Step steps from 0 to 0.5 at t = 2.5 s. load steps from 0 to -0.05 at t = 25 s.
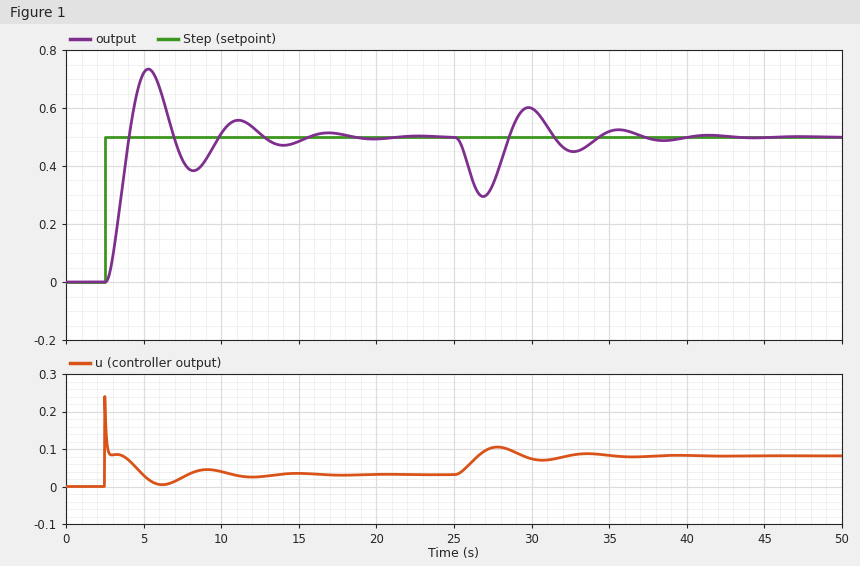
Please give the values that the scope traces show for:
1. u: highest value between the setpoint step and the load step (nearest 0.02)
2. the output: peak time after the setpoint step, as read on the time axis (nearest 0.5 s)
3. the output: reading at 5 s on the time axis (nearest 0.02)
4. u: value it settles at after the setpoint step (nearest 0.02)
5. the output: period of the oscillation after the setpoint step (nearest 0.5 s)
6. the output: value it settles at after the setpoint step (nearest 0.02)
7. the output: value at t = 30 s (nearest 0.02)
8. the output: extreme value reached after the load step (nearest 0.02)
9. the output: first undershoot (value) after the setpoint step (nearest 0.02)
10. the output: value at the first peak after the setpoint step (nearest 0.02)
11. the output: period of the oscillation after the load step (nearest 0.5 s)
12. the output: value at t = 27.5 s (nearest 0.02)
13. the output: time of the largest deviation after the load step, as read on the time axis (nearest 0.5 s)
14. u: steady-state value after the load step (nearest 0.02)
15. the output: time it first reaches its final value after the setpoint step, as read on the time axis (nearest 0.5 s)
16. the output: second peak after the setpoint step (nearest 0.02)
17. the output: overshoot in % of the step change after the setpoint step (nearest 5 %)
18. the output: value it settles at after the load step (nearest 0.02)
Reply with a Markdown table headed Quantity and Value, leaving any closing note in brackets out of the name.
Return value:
| Quantity | Value |
|---|---|
| u: highest value between the setpoint step and the load step | 0.24 |
| the output: peak time after the setpoint step, as read on the time axis | 5.5 s |
| the output: reading at 5 s on the time axis | 0.72 |
| u: value it settles at after the setpoint step | 0.04 |
| the output: period of the oscillation after the setpoint step | 6.0 s |
| the output: value it settles at after the setpoint step | 0.50 |
| the output: value at t = 30 s | 0.60 |
| the output: extreme value reached after the load step | 0.30 |
| the output: first undershoot (value) after the setpoint step | 0.38 |
| the output: value at the first peak after the setpoint step | 0.74 |
| the output: period of the oscillation after the load step | 6.0 s |
| the output: value at t = 27.5 s | 0.34 |
| the output: time of the largest deviation after the load step, as read on the time axis | 27.0 s |
| u: steady-state value after the load step | 0.08 |
| the output: time it first reaches its final value after the setpoint step, as read on the time axis | 4.0 s |
| the output: second peak after the setpoint step | 0.56 |
| the output: overshoot in % of the step change after the setpoint step | 45 % |
| the output: value it settles at after the load step | 0.50 |
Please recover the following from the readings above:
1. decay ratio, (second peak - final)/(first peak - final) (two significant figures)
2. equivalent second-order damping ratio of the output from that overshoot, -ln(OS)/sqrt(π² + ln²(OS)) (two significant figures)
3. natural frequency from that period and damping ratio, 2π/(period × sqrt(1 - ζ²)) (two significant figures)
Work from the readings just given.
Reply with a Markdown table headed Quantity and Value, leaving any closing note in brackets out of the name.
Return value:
| Quantity | Value |
|---|---|
| decay ratio, (second peak - final)/(first peak - final) | 0.25 |
| equivalent second-order damping ratio of the output from that overshoot, -ln(OS)/sqrt(π² + ln²(OS)) | 0.25 |
| natural frequency from that period and damping ratio, 2π/(period × sqrt(1 - ζ²)) | 1.1 rad/s |
